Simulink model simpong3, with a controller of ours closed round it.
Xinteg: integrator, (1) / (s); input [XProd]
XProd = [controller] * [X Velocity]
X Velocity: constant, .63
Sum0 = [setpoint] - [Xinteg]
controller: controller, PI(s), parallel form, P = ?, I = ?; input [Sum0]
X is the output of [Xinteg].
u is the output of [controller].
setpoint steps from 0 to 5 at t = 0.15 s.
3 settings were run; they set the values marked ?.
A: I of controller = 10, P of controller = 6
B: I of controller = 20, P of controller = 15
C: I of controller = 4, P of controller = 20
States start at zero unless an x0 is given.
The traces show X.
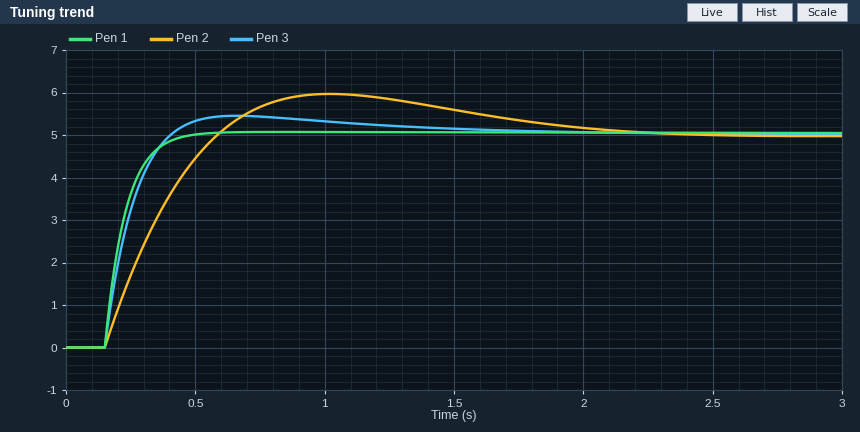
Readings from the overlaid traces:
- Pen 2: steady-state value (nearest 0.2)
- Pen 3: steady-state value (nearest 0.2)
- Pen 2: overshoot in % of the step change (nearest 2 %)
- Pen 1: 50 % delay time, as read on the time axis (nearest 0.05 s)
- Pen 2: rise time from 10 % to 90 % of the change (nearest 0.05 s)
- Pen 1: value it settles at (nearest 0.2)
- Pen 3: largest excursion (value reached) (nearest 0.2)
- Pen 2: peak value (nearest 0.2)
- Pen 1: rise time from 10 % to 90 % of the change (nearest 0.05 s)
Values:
5.0
5.0
20 %
0.20 s
0.35 s
5.0
5.4
6.0
0.15 s
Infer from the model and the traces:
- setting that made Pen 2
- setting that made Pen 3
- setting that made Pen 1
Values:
A
B
C
